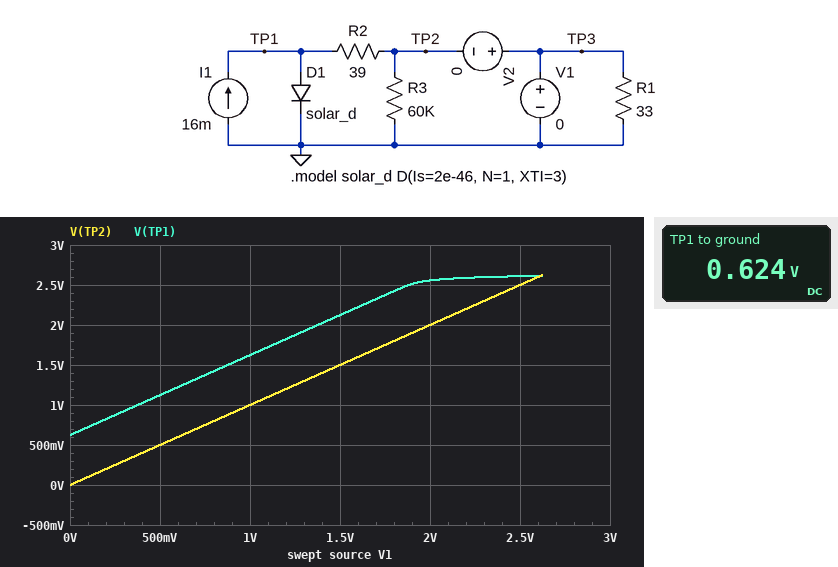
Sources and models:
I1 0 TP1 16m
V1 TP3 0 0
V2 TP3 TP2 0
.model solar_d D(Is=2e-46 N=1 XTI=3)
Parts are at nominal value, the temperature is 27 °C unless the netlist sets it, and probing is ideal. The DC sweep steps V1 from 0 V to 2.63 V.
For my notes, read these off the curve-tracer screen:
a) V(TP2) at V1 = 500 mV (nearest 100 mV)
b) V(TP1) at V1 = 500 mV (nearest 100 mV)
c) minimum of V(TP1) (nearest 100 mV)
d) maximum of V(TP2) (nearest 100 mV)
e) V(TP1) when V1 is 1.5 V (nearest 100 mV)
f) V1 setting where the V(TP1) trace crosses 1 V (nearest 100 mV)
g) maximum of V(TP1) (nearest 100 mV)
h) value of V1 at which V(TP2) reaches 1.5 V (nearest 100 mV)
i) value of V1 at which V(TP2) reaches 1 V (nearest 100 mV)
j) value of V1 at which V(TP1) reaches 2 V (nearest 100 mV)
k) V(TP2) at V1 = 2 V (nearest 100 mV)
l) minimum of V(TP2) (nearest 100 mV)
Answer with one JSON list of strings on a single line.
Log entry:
["500 mV", "1.1 V", "600 mV", "2.6 V", "2.1 V", "400 mV", "2.6 V", "1.5 V", "1.0 V", "1.4 V", "2.0 V", "0 V"]
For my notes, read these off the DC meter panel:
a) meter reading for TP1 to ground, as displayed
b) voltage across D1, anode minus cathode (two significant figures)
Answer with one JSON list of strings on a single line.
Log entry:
["0.624 V", "620 mV"]
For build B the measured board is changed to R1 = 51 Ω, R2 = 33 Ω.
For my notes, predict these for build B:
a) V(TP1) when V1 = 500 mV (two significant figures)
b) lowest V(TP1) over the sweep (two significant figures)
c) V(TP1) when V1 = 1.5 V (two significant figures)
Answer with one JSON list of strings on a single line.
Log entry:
["1.0 V", "530 mV", "2.0 V"]
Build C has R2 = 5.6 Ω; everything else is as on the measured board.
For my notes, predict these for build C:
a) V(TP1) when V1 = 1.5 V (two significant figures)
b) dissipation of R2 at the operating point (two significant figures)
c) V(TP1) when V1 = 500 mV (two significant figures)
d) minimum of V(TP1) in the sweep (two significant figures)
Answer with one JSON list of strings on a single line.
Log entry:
["1.6 V", "1.4 mW", "590 mV", "90 mV"]
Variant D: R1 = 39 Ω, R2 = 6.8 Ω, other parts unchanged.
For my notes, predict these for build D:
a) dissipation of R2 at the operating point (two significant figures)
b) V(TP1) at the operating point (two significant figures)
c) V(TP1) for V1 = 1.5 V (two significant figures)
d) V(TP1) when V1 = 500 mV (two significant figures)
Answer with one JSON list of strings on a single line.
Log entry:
["1.7 mW", "110 mV", "1.6 V", "610 mV"]
